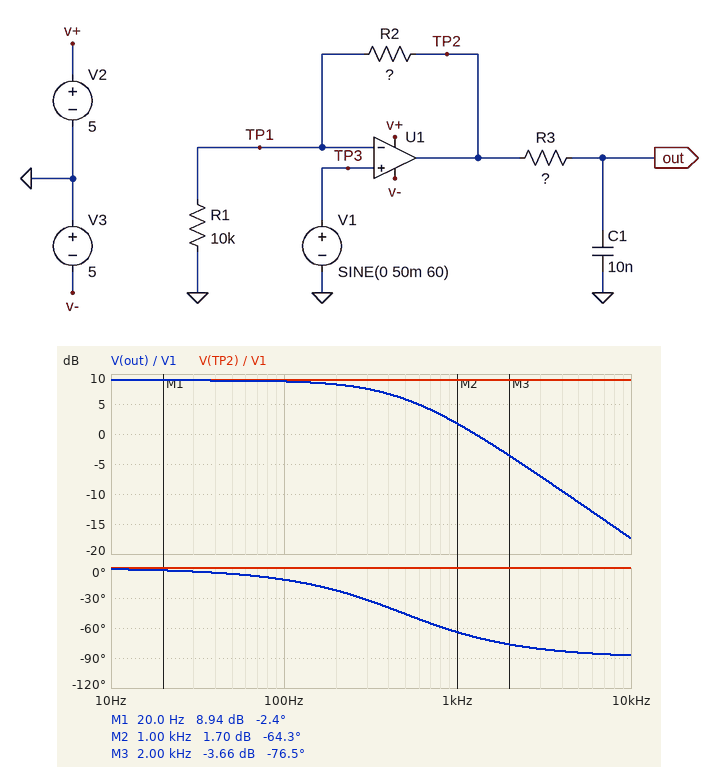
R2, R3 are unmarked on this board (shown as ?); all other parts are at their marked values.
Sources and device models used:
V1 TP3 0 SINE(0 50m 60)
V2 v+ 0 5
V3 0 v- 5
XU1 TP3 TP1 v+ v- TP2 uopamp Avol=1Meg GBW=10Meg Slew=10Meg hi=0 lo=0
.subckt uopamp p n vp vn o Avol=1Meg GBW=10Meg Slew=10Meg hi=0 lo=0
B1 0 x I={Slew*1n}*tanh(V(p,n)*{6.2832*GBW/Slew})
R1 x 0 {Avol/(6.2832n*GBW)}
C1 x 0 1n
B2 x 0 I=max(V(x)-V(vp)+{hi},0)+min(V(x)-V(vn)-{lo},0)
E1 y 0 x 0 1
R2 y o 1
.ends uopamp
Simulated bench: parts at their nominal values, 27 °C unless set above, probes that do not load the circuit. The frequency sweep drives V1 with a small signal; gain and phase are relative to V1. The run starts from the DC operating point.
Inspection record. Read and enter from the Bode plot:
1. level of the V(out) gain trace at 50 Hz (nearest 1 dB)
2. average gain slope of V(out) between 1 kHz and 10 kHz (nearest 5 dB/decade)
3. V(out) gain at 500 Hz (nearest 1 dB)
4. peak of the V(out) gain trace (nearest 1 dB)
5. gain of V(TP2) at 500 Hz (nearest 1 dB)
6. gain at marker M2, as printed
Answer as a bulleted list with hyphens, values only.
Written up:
- 9 dB
- -20 dB/decade
- 6 dB
- 9 dB
- 9 dB
- 1.70 dB
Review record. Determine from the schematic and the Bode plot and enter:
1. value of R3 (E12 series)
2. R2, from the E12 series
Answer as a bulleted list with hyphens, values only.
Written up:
- 33 kΩ
- 18 kΩ
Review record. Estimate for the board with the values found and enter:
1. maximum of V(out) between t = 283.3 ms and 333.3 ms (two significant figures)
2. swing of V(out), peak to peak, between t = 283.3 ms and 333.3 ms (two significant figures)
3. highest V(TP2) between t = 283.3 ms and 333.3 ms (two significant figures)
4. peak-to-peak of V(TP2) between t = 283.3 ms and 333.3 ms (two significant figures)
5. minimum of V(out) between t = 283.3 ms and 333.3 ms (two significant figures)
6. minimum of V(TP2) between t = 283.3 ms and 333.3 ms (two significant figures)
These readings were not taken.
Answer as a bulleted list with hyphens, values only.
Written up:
- 140 mV
- 280 mV
- 140 mV
- 280 mV
- -140 mV
- -140 mV
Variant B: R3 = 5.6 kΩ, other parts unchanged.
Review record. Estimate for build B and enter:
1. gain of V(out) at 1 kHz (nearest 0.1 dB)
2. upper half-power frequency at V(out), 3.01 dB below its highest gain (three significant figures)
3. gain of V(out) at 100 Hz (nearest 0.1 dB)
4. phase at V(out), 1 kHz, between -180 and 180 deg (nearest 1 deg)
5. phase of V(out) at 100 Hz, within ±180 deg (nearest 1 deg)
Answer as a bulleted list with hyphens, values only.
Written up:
- 8.4 dB
- 2.84 kHz
- 8.9 dB
- -19 deg
- -2 deg
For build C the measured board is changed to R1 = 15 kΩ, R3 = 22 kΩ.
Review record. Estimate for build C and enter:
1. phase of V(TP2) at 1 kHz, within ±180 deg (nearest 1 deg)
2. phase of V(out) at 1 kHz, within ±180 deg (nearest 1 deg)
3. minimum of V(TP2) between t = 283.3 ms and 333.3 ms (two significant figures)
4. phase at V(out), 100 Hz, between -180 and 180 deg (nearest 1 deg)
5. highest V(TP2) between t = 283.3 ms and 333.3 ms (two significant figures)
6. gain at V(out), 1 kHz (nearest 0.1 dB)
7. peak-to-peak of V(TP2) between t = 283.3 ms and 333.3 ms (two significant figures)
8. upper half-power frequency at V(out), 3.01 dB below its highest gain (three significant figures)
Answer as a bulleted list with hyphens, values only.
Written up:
- 0 deg
- -54 deg
- -110 mV
- -8 deg
- 110 mV
- 2.2 dB
- 220 mV
- 723 Hz
